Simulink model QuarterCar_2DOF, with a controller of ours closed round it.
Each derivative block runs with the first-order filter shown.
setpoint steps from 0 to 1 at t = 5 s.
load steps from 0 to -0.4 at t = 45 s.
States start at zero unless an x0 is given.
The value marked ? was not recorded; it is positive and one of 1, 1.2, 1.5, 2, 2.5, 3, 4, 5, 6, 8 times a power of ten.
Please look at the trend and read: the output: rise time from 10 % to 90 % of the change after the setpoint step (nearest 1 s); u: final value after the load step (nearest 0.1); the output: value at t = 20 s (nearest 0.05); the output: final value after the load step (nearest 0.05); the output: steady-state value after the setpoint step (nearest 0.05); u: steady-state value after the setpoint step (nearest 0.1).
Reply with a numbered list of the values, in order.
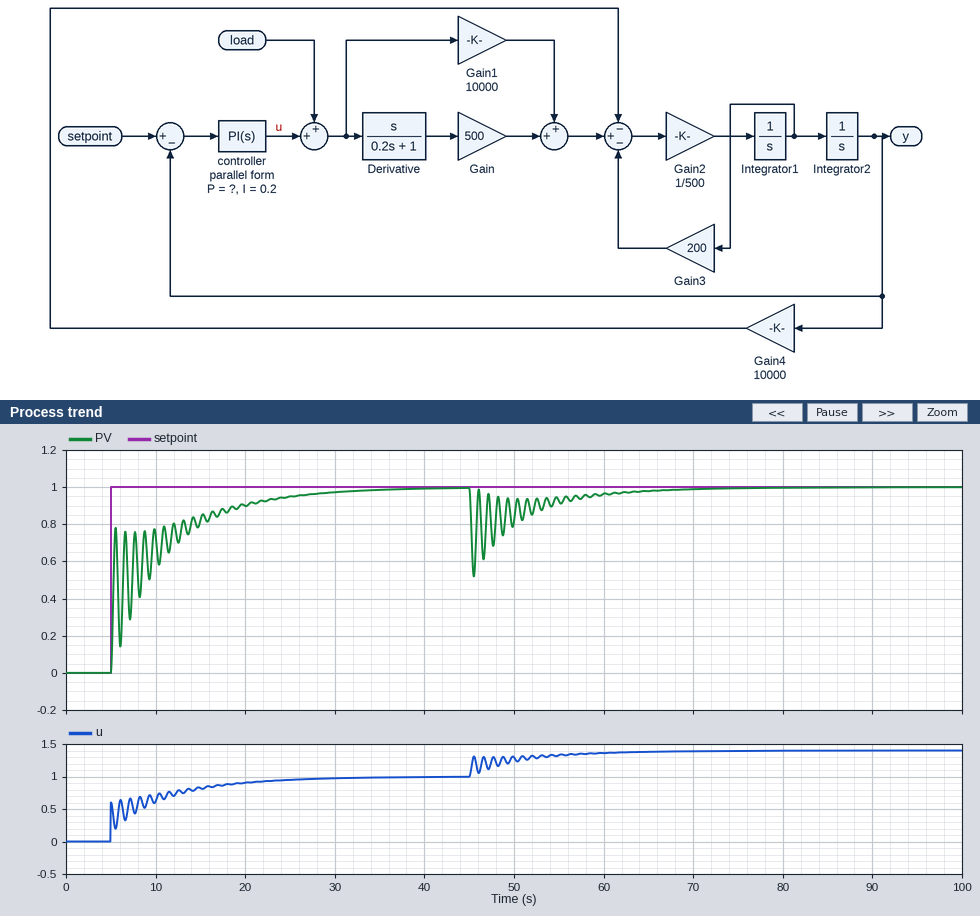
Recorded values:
1. 14 s
2. 1.4
3. 0.90
4. 1.00
5. 1.00
6. 1.0
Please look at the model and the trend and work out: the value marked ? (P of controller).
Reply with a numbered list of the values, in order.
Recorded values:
1. 0.6
